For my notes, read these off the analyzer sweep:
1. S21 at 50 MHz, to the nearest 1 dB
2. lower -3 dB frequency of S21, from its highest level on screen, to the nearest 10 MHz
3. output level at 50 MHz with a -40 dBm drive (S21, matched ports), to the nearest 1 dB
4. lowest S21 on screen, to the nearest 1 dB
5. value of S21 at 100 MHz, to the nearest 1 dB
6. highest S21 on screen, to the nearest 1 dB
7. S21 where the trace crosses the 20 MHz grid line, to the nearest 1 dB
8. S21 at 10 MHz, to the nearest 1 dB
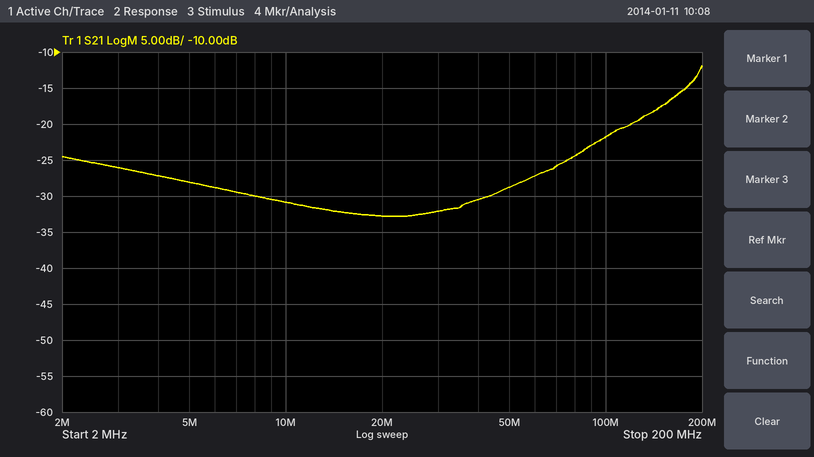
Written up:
-29 dB
180 MHz
-69 dBm
-33 dB
-22 dB
-12 dB
-33 dB
-31 dB
